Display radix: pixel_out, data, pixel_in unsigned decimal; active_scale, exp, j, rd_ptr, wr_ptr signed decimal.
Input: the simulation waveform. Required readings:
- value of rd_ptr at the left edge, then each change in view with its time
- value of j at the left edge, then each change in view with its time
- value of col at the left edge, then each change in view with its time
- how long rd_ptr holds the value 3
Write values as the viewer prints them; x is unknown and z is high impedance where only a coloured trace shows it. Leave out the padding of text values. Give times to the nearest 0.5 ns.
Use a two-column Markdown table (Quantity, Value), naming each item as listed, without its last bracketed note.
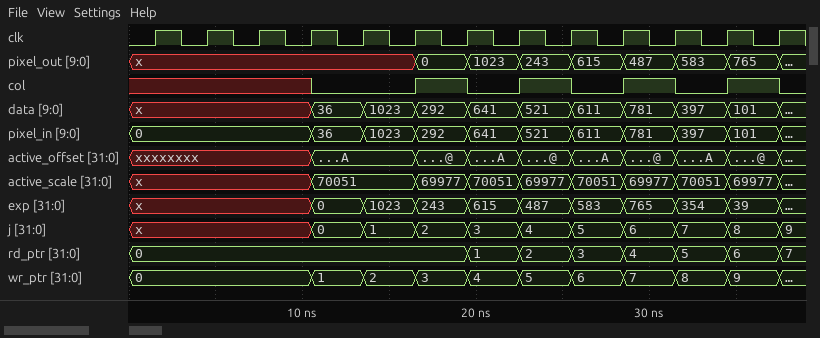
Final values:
| Quantity | Value |
|---|---|
| value of rd_ptr at the left edge, then each change in view with its time | 0, 1 at 19.5 ns, 2 at 22.5 ns, 3 at 25.5 ns, 4 at 28.5 ns, 5 at 31.5 ns, 6 at 34.5 ns, 7 at 37.5 ns |
| value of j at the left edge, then each change in view with its time | x, 0 at 10.5 ns, 1 at 13.5 ns, 2 at 16.5 ns, 3 at 19.5 ns, 4 at 22.5 ns, 5 at 25.5 ns, 6 at 28.5 ns, 7 at 31.5 ns, 8 at 34.5 ns, 9 at 37.5 ns |
| value of col at the left edge, then each change in view with its time | x, 0 at 10.5 ns, 1 at 16.5 ns, 0 at 19.5 ns, 1 at 22.5 ns, 0 at 25.5 ns, 1 at 28.5 ns, 0 at 31.5 ns, 1 at 34.5 ns, 0 at 37.5 ns |
| how long rd_ptr holds the value 3 | 3 ns |
